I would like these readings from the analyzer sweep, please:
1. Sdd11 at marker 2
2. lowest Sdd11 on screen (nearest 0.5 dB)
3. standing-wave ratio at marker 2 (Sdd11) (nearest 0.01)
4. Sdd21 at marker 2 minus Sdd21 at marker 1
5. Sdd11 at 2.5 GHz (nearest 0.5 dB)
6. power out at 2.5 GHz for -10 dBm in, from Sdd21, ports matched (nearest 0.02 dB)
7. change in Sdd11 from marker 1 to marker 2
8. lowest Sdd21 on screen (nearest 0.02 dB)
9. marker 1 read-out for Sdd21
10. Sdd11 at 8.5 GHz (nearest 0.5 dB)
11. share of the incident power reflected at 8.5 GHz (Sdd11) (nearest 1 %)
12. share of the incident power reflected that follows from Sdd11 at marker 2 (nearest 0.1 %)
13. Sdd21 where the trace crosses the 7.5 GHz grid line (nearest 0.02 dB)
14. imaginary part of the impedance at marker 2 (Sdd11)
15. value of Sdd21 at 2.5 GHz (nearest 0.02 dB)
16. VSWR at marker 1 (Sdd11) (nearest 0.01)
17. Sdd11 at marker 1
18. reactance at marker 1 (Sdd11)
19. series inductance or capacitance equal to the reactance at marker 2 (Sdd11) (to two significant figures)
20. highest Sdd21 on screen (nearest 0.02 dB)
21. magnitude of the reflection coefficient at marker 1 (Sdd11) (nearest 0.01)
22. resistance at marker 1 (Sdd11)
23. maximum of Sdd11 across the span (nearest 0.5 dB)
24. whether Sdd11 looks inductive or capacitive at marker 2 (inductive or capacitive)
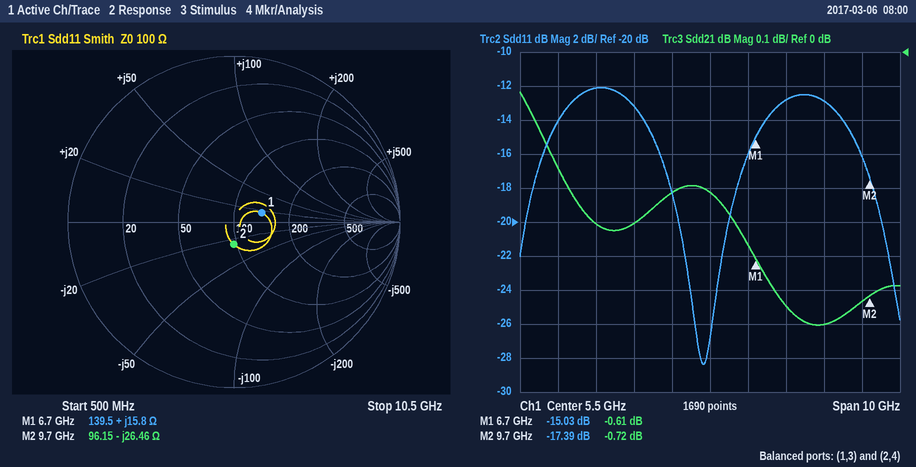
-17.39 dB
-28.5 dB
1.31
-0.11 dB
-12.0 dB
-10.50 dBm
-2.36 dB
-0.80 dB
-0.61 dB
-13.0 dB
5 %
1.8 %
-0.74 dB
-26.46 Ω
-0.50 dB
1.43
-15.03 dB
+15.8 Ω
620 fF
-0.12 dB
0.18
139.5 Ω
-12.0 dB
capacitive
